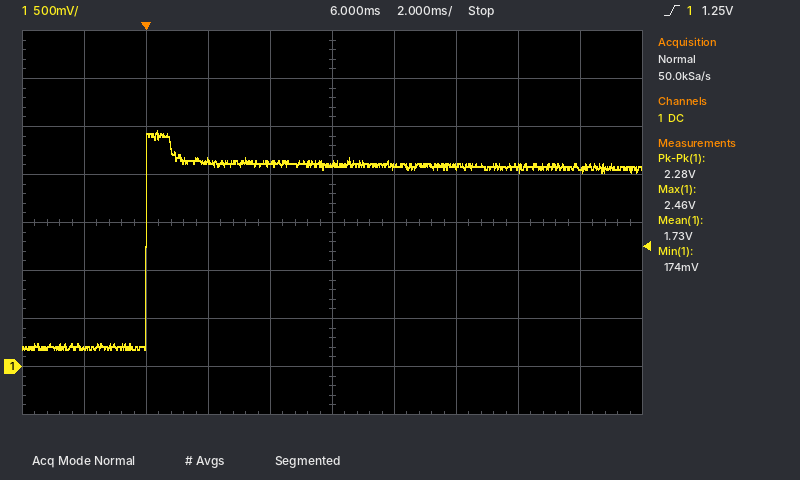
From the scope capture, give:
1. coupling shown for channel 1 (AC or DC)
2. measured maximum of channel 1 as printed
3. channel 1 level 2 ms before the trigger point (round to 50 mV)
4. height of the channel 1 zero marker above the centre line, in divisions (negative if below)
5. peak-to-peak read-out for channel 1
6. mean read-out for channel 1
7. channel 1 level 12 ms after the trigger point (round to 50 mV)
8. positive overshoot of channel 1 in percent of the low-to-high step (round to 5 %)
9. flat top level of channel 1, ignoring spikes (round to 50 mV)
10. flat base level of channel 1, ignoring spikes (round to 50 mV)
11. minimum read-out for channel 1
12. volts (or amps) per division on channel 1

DC
2.46 V
200 mV
-3.0 div
2.28 V
1.73 V
2.05 V
20 %
2.10 V
200 mV
174 mV
500 mV
